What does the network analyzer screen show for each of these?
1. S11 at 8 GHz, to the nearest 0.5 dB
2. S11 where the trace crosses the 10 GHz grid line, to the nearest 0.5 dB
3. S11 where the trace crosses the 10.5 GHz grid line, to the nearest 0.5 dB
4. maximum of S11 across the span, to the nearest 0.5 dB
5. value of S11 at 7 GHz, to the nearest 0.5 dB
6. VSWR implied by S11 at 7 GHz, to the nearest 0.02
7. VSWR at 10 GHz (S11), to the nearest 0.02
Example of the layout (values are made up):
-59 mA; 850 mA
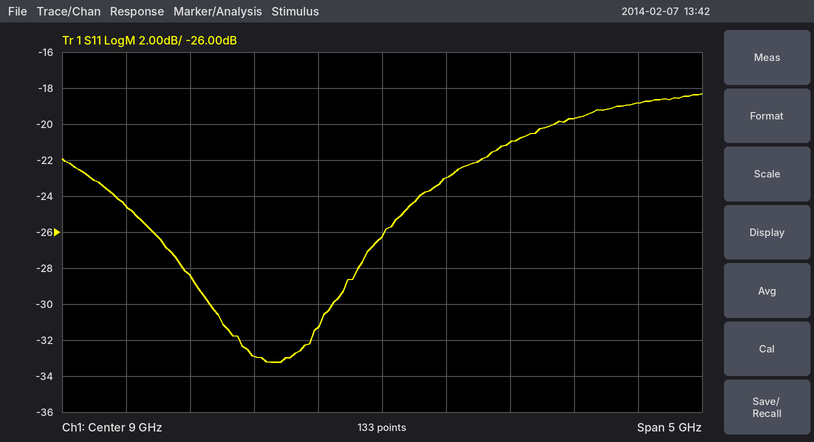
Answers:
-33.0 dB; -21.0 dB; -19.5 dB; -18.5 dB; -24.5 dB; 1.12; 1.20
